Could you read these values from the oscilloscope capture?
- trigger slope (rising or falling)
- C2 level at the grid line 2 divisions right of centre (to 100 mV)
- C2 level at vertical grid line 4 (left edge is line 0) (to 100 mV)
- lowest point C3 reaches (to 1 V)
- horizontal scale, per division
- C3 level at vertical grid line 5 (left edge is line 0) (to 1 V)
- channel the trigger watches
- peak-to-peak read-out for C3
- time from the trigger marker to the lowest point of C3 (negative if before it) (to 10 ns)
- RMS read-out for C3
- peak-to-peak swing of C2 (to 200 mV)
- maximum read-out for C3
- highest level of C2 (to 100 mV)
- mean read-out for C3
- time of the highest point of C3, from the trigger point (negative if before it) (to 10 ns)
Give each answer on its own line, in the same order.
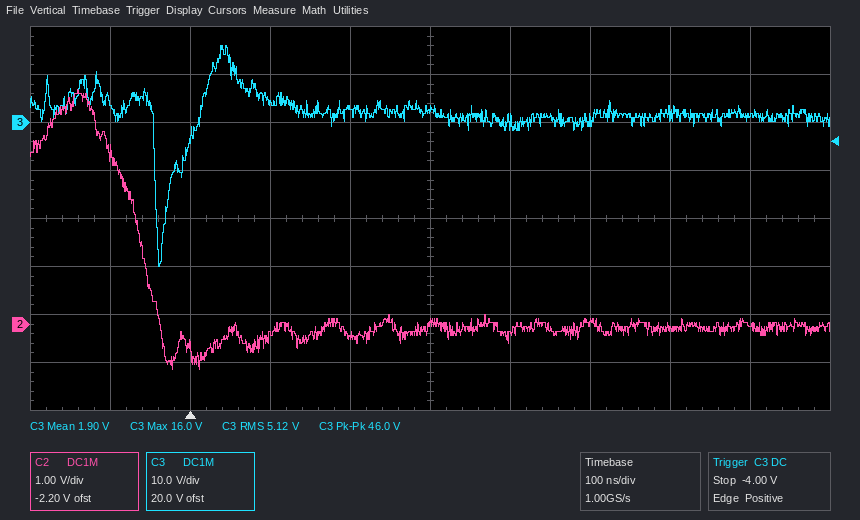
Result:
rising
0.0 V
-200 mV
-30 V
100 ns
3 V
C3
46.0 V
-40 ns
5.12 V
5.8 V
16.0 V
4.9 V
1.90 V
+40 ns
